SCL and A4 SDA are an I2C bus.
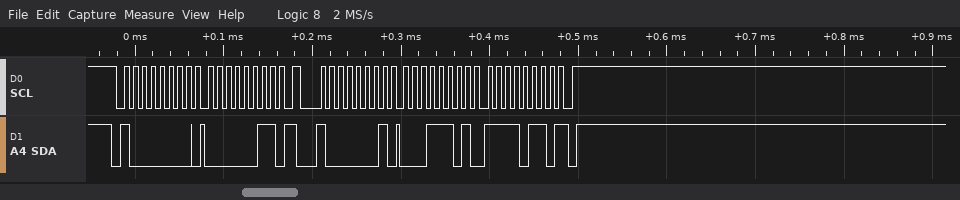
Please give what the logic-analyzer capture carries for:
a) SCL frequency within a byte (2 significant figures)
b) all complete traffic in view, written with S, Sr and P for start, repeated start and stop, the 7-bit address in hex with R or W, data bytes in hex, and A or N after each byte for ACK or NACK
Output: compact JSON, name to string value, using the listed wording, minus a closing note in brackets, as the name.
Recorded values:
{"SCL frequency within a byte": "100 kHz", "all complete traffic in view, written with S, Sr and P for start, repeated start and stop, the 7-bit address in hex with R or W, data bytes in hex, and A or N after each byte for ACK or NACK": "S 40W A 03 A Sr 40R A 1D A F6 N P"}
